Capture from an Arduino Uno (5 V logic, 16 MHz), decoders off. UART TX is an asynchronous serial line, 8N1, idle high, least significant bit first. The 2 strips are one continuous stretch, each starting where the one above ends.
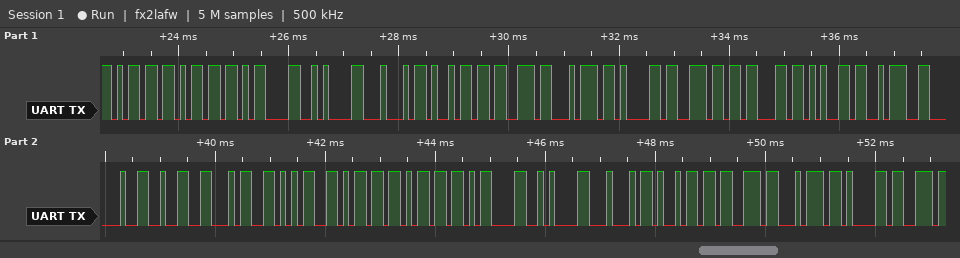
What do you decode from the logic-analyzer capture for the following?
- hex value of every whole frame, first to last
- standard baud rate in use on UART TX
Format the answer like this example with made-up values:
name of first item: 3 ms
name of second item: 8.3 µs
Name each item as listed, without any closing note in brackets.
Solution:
hex value of every whole frame, first to last: 0x6D 0x6D 0x0D 0x0A 0x44 0x69 0x73 0x74 0x61 0x6E 0x63 0x65 0x3A 0x20 0x32 0x34 0x35 0x6D 0x6D 0x0D 0x0A 0x44 0x69 0x73 0x74 0x61
standard baud rate in use on UART TX: 9600 baud
